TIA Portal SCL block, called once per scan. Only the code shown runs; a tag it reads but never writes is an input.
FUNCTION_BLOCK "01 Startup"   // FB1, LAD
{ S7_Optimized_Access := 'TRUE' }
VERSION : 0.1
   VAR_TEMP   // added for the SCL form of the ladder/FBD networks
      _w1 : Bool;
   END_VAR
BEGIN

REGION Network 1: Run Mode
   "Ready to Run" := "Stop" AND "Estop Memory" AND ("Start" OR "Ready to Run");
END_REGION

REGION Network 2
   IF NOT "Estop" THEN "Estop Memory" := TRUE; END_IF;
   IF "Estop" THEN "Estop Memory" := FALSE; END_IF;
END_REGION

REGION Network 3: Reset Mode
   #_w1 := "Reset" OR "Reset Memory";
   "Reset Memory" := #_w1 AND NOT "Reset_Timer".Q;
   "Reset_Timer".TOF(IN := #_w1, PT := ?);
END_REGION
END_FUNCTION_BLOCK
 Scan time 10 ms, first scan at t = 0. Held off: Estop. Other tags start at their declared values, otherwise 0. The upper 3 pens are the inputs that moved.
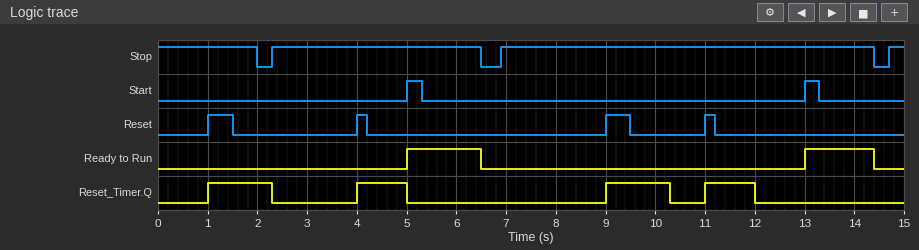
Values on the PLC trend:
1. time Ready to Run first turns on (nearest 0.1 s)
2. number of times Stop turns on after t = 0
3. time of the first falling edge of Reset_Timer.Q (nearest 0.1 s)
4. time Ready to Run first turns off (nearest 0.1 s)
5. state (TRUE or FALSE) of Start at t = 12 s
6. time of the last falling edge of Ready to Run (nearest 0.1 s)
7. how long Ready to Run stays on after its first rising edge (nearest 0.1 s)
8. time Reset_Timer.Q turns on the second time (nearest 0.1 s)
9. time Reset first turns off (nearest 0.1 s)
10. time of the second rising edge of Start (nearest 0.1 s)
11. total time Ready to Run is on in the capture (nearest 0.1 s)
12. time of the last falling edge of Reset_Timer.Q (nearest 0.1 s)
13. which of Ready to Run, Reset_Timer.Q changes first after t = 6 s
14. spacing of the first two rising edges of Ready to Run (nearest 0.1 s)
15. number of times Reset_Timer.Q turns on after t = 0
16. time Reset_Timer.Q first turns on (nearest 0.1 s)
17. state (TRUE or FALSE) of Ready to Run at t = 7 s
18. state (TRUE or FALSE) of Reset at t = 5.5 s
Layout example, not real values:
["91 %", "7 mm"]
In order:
["5.0 s", "3", "2.3 s", "6.5 s", "FALSE", "14.4 s", "1.5 s", "4.0 s", "1.5 s", "13.0 s", "2.9 s", "12.0 s", "Ready to Run", "8.0 s", "4", "1.0 s", "FALSE", "FALSE"]
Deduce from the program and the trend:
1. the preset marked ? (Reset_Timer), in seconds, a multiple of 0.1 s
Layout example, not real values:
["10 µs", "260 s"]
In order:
["0.8 s"]
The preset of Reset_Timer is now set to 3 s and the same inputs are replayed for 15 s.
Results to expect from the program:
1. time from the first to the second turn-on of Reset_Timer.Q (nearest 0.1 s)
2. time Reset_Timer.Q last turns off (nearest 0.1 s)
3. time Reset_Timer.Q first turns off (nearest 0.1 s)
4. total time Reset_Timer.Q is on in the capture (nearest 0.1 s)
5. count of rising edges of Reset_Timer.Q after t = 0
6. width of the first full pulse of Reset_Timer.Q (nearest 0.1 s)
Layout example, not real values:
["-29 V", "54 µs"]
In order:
["8.0 s", "14.2 s", "7.2 s", "11.4 s", "2", "6.2 s"]
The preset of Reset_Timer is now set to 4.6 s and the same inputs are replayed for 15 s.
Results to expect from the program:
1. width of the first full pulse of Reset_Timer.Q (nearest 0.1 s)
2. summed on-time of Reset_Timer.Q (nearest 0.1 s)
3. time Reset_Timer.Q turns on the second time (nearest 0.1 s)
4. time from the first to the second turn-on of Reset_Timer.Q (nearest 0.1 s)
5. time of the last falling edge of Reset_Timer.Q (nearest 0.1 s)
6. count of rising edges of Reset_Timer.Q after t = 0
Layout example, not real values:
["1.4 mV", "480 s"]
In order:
["7.8 s", "13.8 s", "9.0 s", "8.0 s", "8.8 s", "2"]
